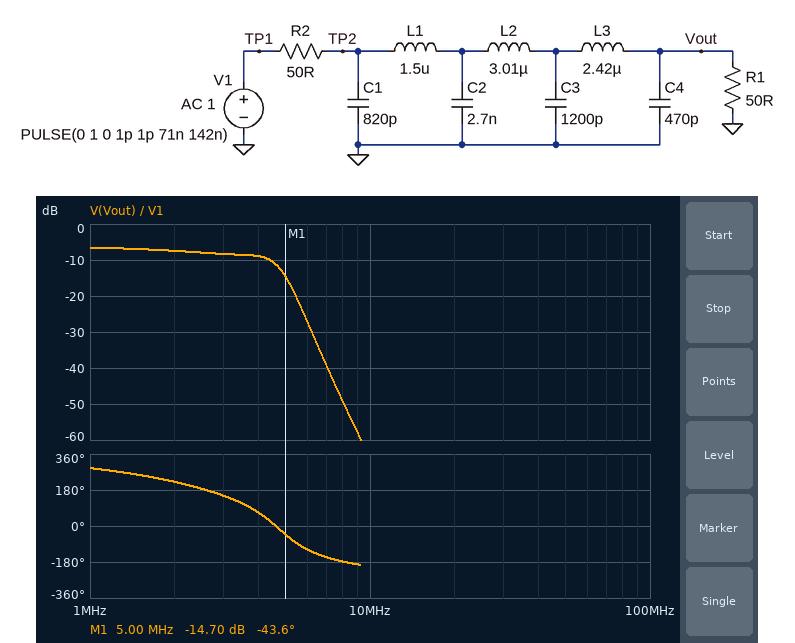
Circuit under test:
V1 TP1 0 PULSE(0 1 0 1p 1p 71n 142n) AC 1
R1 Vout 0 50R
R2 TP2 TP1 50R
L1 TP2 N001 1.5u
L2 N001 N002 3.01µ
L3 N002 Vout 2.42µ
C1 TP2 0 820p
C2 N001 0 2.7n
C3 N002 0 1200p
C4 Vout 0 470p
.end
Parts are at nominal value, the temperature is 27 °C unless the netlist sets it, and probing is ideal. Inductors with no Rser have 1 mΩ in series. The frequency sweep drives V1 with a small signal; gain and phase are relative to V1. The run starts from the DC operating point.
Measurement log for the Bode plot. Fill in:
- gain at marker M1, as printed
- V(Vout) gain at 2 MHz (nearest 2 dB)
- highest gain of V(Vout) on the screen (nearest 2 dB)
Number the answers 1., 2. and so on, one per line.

1. -14.70 dB
2. -8 dB
3. -6 dB
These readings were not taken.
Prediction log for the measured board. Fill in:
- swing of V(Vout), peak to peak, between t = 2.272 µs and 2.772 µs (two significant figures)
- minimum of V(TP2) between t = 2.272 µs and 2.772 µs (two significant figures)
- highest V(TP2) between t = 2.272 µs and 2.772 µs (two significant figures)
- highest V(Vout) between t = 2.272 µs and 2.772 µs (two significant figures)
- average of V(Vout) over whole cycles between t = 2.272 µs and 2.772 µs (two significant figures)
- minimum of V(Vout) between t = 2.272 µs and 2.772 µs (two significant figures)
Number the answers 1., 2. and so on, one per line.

1. 13 mV
2. -190 mV
3. 690 mV
4. 260 mV
5. 250 mV
6. 240 mV
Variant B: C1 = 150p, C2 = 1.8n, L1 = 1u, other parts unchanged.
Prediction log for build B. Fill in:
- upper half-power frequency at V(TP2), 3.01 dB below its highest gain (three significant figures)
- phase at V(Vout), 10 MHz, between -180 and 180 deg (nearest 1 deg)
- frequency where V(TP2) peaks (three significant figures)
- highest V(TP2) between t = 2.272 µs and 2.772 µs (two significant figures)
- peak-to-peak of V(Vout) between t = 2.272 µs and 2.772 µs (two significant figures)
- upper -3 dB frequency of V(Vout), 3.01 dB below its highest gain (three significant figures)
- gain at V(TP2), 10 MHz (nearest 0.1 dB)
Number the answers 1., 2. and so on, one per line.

1. 27.5 MHz
2. -113 deg
3. 13.5 MHz
4. 860 mV
5. 32 mV
6. 4.37 MHz
7. -0.8 dB
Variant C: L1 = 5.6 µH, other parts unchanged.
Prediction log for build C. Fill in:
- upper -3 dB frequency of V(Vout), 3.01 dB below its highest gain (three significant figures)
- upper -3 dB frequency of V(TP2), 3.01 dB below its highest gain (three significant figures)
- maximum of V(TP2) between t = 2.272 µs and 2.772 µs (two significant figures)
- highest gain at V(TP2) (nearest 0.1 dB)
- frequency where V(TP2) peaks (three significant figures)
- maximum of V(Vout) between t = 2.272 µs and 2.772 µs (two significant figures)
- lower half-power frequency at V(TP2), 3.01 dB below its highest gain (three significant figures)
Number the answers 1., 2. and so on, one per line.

1. 2.42 MHz
2. 5.54 MHz
3. 620 mV
4. -0.7 dB
5. 3.03 MHz
6. 250 mV
7. 1.92 MHz
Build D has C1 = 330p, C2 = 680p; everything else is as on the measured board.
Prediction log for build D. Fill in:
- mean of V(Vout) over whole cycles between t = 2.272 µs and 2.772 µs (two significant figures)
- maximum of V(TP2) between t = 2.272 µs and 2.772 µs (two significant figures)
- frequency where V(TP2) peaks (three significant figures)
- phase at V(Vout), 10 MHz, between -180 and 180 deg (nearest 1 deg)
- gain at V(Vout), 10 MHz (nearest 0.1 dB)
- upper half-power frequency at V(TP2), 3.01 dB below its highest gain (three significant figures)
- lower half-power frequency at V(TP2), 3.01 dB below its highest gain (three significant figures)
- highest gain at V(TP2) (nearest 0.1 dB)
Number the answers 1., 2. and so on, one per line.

1. 250 mV
2. 630 mV
3. 9.01 MHz
4. -154 deg
5. -43.0 dB
6. 13.9 MHz
7. 7.49 MHz
8. 0 dB
